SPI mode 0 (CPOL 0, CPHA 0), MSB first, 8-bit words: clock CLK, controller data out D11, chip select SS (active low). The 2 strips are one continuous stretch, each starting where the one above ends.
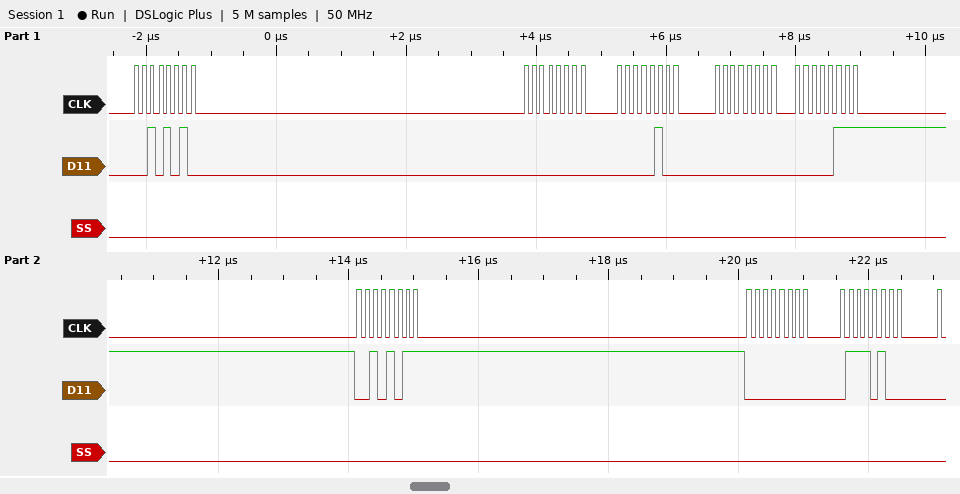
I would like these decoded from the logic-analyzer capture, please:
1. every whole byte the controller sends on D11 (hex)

2A 00 04 00 07 2B 00 74
